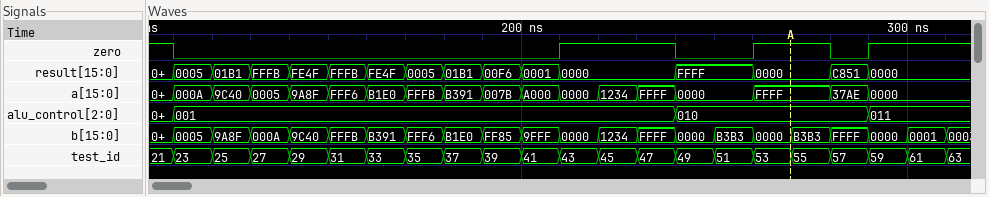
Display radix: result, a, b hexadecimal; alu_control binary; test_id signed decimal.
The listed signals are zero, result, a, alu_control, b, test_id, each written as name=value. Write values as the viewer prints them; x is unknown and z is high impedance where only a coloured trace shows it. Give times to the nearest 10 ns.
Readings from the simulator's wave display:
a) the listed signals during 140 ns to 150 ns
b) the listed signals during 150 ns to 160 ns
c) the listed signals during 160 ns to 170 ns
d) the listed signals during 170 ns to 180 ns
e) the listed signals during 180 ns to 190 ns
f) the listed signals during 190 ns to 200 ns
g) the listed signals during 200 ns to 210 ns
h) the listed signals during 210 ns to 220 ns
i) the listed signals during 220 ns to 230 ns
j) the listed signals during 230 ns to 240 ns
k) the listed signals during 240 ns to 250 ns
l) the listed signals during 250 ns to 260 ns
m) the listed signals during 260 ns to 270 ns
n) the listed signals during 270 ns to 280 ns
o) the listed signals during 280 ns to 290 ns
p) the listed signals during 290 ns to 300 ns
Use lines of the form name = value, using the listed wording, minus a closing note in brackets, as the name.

the listed signals during 140 ns to 150 ns = zero=0, result=FE4F, a=9A8F, alu_control=001, b=9C40, test_id=29
the listed signals during 150 ns to 160 ns = zero=0, result=FFFB, a=FFF6, alu_control=001, b=FFFB, test_id=31
the listed signals during 160 ns to 170 ns = zero=0, result=FE4F, a=B1E0, alu_control=001, b=B391, test_id=33
the listed signals during 170 ns to 180 ns = zero=0, result=0005, a=FFFB, alu_control=001, b=FFF6, test_id=35
the listed signals during 180 ns to 190 ns = zero=0, result=01B1, a=B391, alu_control=001, b=B1E0, test_id=37
the listed signals during 190 ns to 200 ns = zero=0, result=00F6, a=007B, alu_control=001, b=FF85, test_id=39
the listed signals during 200 ns to 210 ns = zero=0, result=0001, a=A000, alu_control=001, b=9FFF, test_id=41
the listed signals during 210 ns to 220 ns = zero=1, result=0000, a=0000, alu_control=001, b=0000, test_id=43
the listed signals during 220 ns to 230 ns = zero=1, result=0000, a=1234, alu_control=001, b=1234, test_id=45
the listed signals during 230 ns to 240 ns = zero=1, result=0000, a=FFFF, alu_control=001, b=FFFF, test_id=47
the listed signals during 240 ns to 250 ns = zero=0, result=FFFF, a=0000, alu_control=010, b=0000, test_id=49
the listed signals during 250 ns to 260 ns = zero=0, result=FFFF, a=0000, alu_control=010, b=B3B3, test_id=51
the listed signals during 260 ns to 270 ns = zero=1, result=0000, a=FFFF, alu_control=010, b=0000, test_id=53
the listed signals during 270 ns to 280 ns = zero=1, result=0000, a=FFFF, alu_control=010, b=B3B3, test_id=55
the listed signals during 280 ns to 290 ns = zero=0, result=C851, a=37AE, alu_control=010, b=FFFF, test_id=57
the listed signals during 290 ns to 300 ns = zero=1, result=0000, a=0000, alu_control=011, b=0000, test_id=59
